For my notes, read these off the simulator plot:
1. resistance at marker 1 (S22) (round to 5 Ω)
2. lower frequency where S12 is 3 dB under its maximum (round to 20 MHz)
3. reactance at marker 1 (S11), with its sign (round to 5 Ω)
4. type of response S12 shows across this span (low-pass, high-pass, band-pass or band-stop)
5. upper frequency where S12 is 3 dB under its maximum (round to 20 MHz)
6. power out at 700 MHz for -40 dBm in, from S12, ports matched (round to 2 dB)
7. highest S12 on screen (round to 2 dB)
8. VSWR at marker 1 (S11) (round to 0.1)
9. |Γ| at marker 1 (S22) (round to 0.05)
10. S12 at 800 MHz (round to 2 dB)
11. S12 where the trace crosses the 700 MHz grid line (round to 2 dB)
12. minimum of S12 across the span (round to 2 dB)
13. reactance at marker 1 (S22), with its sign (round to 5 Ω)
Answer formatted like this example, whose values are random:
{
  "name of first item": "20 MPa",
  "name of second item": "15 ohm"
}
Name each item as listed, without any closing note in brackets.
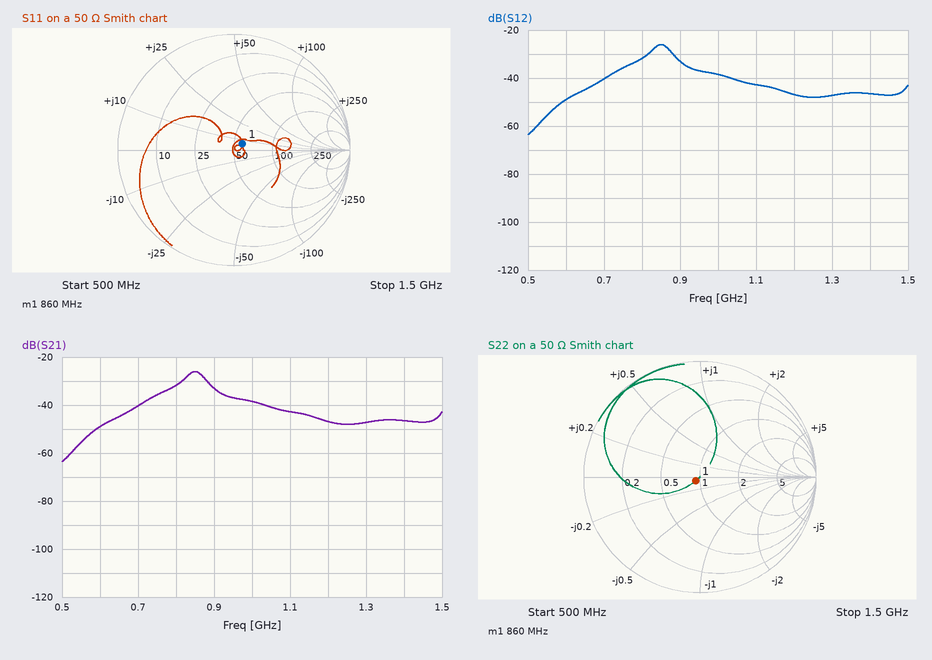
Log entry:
{
  "resistance at marker 1 (S22)": "45 Ω",
  "lower frequency where S12 is 3 dB under its maximum": "820 MHz",
  "reactance at marker 1 (S11), with its sign": "+5 Ω",
  "type of response S12 shows across this span": "band-pass",
  "upper frequency where S12 is 3 dB under its maximum": "880 MHz",
  "power out at 700 MHz for -40 dBm in, from S12, ports matched": "-80 dBm",
  "highest S12 on screen": "-26 dB",
  "VSWR at marker 1 (S11)": "1.2",
  "|Γ| at marker 1 (S22)": "0.05",
  "S12 at 800 MHz": "-32 dB",
  "S12 where the trace crosses the 700 MHz grid line": "-40 dB",
  "minimum of S12 across the span": "-64 dB",
  "reactance at marker 1 (S22), with its sign": "-5 Ω"
}
